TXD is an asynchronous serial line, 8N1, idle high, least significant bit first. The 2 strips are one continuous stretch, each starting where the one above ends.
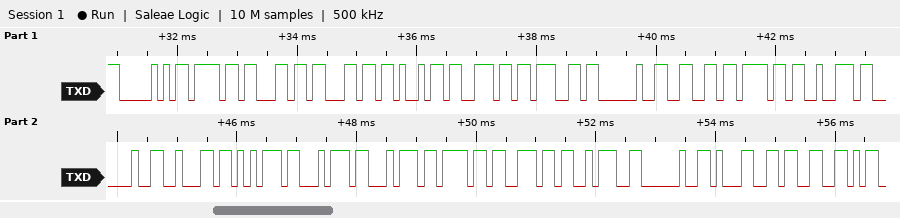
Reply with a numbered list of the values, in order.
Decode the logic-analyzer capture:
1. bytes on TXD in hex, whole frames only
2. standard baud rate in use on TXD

1. 50 6F 6C 6C 69 6E 67 20 66 6F 72 20 62 75 74 74 6F 6E 3A 20 31 33
2. 9600 baud
